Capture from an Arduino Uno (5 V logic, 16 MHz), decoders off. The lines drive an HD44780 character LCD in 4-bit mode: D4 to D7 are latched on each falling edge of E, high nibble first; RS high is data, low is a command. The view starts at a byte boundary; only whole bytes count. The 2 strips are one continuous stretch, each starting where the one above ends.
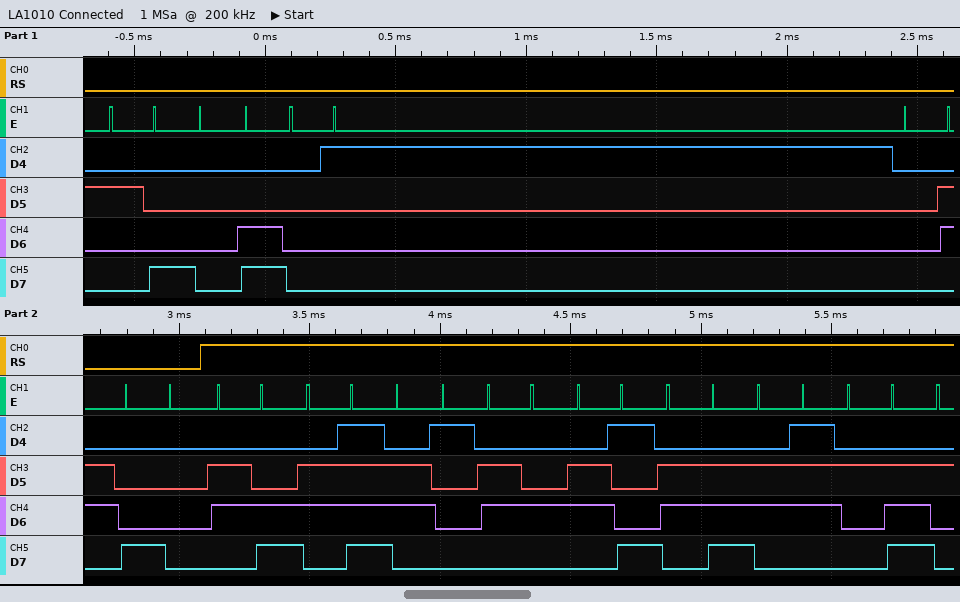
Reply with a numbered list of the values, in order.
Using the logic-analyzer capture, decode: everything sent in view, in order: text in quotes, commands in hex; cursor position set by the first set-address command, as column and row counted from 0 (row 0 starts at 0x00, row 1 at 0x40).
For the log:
1. 0x28 0x0C 0x01 0x06 0x80 "loading."
2. column 0, row 0
